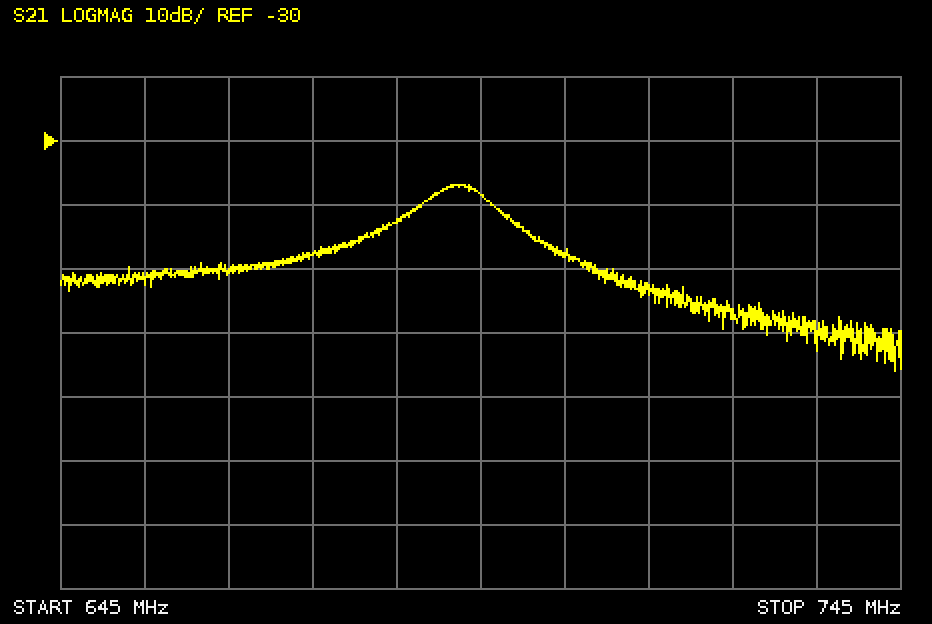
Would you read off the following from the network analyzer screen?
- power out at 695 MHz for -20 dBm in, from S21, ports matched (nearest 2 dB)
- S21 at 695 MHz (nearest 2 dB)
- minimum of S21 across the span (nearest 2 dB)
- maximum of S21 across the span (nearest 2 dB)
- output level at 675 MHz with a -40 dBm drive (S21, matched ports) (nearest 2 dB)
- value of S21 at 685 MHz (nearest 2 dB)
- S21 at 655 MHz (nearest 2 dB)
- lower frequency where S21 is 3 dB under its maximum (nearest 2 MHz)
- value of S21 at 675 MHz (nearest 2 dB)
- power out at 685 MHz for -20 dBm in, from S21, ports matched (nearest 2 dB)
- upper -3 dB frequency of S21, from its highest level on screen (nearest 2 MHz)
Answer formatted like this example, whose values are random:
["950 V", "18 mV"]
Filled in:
["-58 dBm", "-38 dB", "-66 dB", "-36 dB", "-88 dBm", "-42 dB", "-52 dB", "688 MHz", "-48 dB", "-62 dBm", "696 MHz"]
